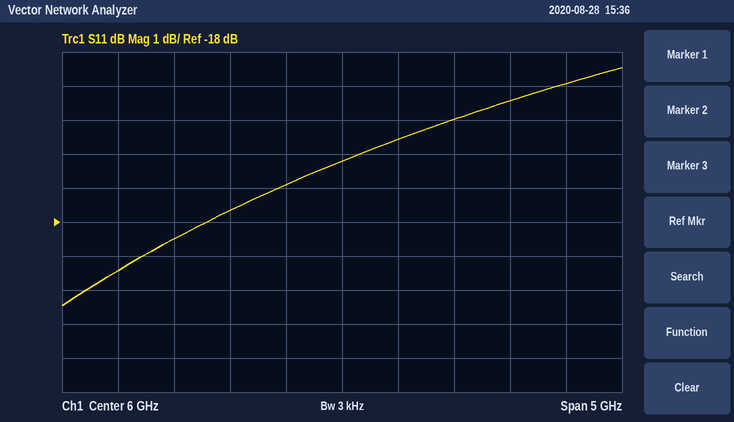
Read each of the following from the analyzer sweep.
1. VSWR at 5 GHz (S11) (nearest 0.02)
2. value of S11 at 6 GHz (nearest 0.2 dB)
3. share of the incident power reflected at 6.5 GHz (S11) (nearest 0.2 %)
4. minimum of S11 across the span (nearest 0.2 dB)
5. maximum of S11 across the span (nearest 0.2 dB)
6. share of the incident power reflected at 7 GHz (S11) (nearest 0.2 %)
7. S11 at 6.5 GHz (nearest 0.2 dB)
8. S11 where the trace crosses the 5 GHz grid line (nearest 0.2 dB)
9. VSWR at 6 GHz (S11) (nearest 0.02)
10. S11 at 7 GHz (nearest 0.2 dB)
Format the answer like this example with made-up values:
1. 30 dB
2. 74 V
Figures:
1. 1.30
2. -16.2 dB
3. 2.8 %
4. -20.4 dB
5. -13.4 dB
6. 3.2 %
7. -15.6 dB
8. -17.6 dB
9. 1.36
10. -15.0 dB
